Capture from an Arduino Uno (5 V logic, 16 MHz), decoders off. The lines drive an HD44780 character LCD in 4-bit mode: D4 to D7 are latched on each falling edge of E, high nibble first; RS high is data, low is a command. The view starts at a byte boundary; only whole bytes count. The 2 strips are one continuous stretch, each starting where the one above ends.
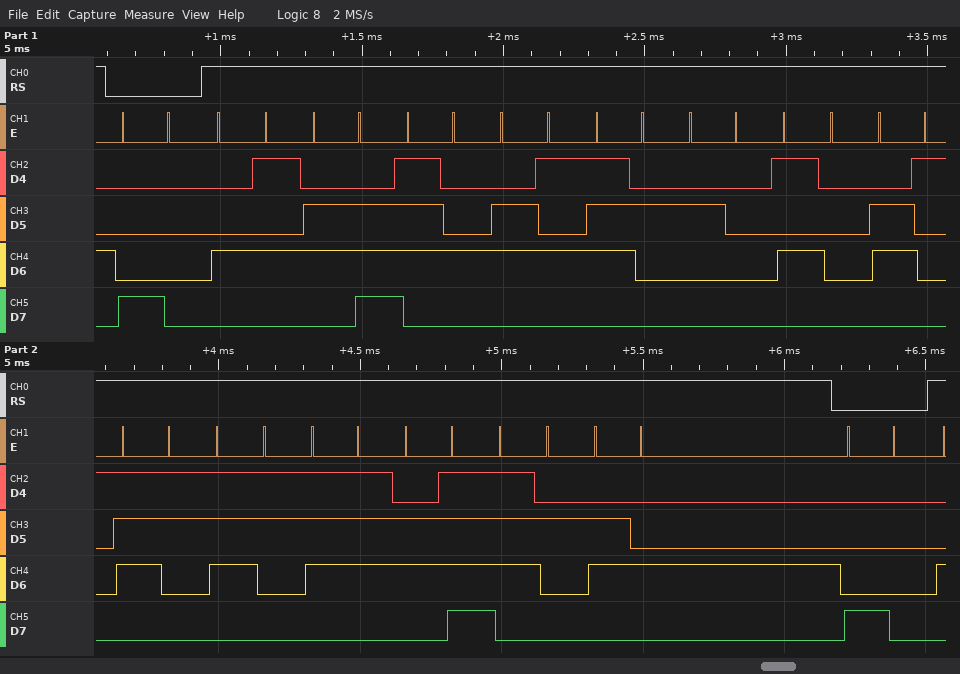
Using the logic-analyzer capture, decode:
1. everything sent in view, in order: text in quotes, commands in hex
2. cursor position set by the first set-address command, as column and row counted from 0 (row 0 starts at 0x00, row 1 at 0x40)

0x80 "Enter Password" 0x80
column 0, row 0
